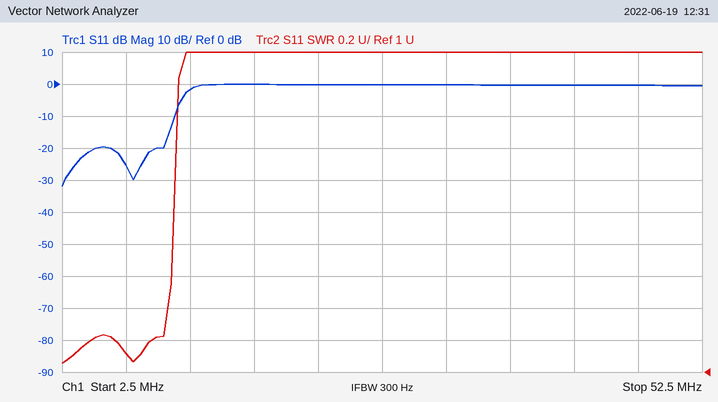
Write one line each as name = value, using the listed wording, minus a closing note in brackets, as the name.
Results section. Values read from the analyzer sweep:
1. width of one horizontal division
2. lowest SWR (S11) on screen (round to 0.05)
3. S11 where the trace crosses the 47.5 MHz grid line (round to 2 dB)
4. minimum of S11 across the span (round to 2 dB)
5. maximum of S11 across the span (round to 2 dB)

width of one horizontal division = 5 MHz
lowest SWR (S11) on screen = 1.05
S11 where the trace crosses the 47.5 MHz grid line = 0 dB
minimum of S11 across the span = -32 dB
maximum of S11 across the span = 0 dB
